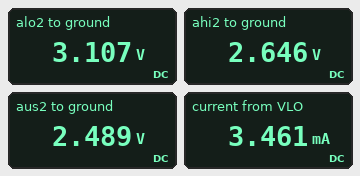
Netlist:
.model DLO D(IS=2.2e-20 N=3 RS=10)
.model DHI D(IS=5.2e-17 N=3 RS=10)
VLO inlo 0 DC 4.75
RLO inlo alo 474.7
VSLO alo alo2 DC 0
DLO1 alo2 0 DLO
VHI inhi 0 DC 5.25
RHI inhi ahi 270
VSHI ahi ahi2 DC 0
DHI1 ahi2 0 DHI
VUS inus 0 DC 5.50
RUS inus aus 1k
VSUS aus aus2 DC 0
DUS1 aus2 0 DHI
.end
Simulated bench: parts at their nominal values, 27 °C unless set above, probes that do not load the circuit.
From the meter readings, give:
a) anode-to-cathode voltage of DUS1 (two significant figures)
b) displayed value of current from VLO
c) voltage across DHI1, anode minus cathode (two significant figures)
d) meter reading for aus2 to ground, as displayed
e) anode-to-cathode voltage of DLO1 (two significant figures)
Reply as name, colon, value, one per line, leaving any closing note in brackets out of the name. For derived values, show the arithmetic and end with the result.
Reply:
anode-to-cathode voltage of DUS1: 2.489 V = 2.5 V
displayed value of current from VLO: 3.461 mA
voltage across DHI1, anode minus cathode: 2.646 V = 2.6 V
meter reading for aus2 to ground, as displayed: 2.489 V
anode-to-cathode voltage of DLO1: 3.107 V = 3.1 V
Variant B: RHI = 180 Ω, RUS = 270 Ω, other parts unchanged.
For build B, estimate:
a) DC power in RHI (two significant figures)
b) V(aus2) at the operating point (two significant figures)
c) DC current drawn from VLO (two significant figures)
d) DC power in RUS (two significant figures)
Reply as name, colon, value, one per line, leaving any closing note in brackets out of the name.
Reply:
DC power in RHI: 36 mW
V(aus2) at the operating point: 2.7 V
DC current drawn from VLO: 3.5 mA
DC power in RUS: 30 mW
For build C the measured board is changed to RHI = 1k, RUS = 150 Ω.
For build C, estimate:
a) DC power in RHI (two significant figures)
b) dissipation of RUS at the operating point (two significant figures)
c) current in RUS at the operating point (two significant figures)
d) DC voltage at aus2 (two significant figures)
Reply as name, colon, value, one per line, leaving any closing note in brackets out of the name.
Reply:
DC power in RHI: 7.7 mW
dissipation of RUS at the operating point: 49 mW
current in RUS at the operating point: 18 mA
DC voltage at aus2: 2.8 V
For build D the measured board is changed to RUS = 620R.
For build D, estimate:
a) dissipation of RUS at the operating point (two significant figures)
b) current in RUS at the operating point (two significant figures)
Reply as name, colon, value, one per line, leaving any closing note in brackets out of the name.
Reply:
dissipation of RUS at the operating point: 14 mW
current in RUS at the operating point: 4.8 mA
